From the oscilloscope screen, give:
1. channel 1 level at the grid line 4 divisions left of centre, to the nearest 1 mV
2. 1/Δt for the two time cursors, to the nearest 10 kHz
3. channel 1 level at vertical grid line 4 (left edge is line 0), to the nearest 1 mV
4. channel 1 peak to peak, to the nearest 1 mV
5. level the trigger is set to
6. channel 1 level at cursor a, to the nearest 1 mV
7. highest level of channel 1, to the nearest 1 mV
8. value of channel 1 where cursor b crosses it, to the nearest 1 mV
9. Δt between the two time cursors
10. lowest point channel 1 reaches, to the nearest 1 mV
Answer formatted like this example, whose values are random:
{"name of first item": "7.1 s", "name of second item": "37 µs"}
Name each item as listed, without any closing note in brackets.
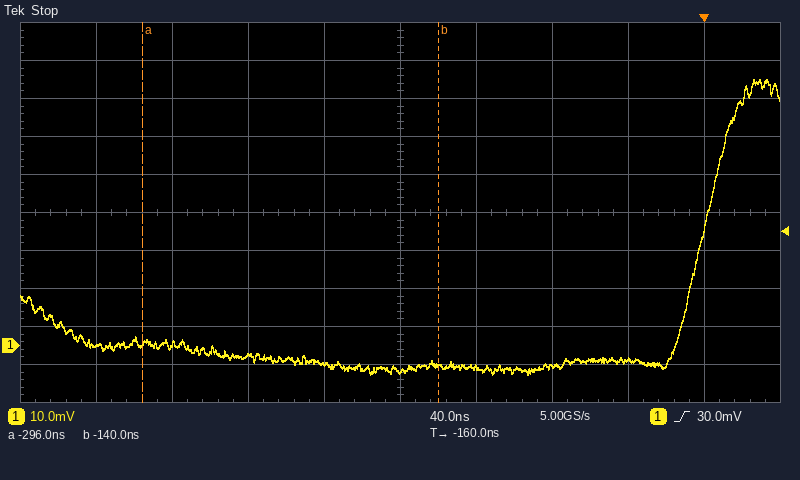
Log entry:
{"channel 1 level at the grid line 4 divisions left of centre, to the nearest 1 mV": "0 mV", "1/Δt for the two time cursors, to the nearest 10 kHz": "6.41 MHz", "channel 1 level at vertical grid line 4 (left edge is line 0), to the nearest 1 mV": "-5 mV", "channel 1 peak to peak, to the nearest 1 mV": "78 mV", "level the trigger is set to": "30.0 mV", "channel 1 level at cursor a, to the nearest 1 mV": "0 mV", "highest level of channel 1, to the nearest 1 mV": "70 mV", "value of channel 1 where cursor b crosses it, to the nearest 1 mV": "-5 mV", "Δt between the two time cursors": "156 ns", "lowest point channel 1 reaches, to the nearest 1 mV": "-8 mV"}
